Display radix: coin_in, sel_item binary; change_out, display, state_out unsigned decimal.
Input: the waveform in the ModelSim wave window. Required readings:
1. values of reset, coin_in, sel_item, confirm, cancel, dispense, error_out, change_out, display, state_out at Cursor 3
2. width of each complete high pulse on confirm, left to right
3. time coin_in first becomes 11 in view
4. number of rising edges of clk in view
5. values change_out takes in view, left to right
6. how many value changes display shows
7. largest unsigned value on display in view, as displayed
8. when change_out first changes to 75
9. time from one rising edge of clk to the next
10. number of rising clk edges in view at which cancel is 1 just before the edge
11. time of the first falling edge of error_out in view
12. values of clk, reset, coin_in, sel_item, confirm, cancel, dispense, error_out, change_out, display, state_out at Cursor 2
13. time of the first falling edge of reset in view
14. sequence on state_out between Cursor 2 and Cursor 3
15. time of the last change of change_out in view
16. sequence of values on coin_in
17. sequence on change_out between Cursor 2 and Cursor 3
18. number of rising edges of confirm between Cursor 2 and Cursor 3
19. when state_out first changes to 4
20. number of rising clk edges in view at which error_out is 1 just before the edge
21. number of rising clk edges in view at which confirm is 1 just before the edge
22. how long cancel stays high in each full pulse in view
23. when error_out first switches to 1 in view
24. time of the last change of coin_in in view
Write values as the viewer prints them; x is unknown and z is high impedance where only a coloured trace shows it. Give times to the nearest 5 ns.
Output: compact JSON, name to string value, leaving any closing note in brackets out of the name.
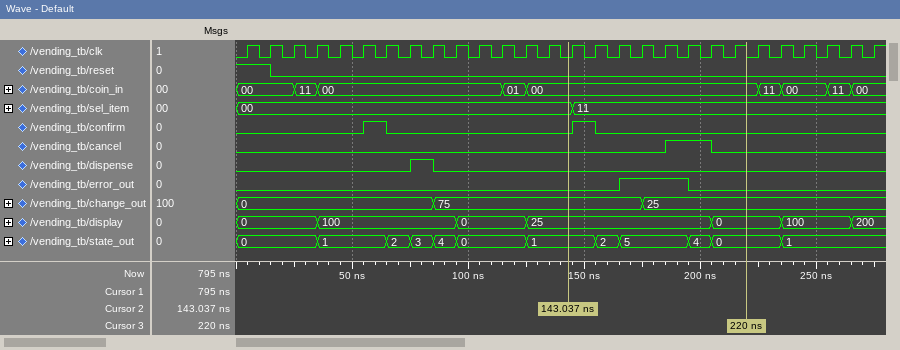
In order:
{"values of reset, coin_in, sel_item, confirm, cancel, dispense, error_out, change_out, display, state_out at Cursor 3": "reset=0, coin_in=00, sel_item=11, confirm=0, cancel=0, dispense=0, error_out=0, change_out=25, display=0, state_out=0", "width of each complete high pulse on confirm, left to right": "10 ns, 10 ns", "time coin_in first becomes 11 in view": "25 ns", "number of rising edges of clk in view": "28", "values change_out takes in view, left to right": "0, 75, 25", "how many value changes display shows": "6", "largest unsigned value on display in view, as displayed": "200", "when change_out first changes to 75": "85 ns", "time from one rising edge of clk to the next": "10 ns", "number of rising clk edges in view at which cancel is 1 just before the edge": "2", "time of the first falling edge of error_out in view": "195 ns", "values of clk, reset, coin_in, sel_item, confirm, cancel, dispense, error_out, change_out, display, state_out at Cursor 2": "clk=0, reset=0, coin_in=00, sel_item=00, confirm=0, cancel=0, dispense=0, error_out=0, change_out=75, display=25, state_out=1", "time of the first falling edge of reset in view": "15 ns", "sequence on state_out between Cursor 2 and Cursor 3": "1, 2, 5, 4, 0", "time of the last change of change_out in view": "175 ns", "sequence of values on coin_in": "00, 11, 00, 01, 00, 11, 00, 11, 00", "sequence on change_out between Cursor 2 and Cursor 3": "75, 25", "number of rising edges of confirm between Cursor 2 and Cursor 3": "1", "when state_out first changes to 4": "85 ns", "number of rising clk edges in view at which error_out is 1 just before the edge": "3", "number of rising clk edges in view at which confirm is 1 just before the edge": "2", "how long cancel stays high in each full pulse in view": "20 ns", "when error_out first switches to 1 in view": "165 ns", "time of the last change of coin_in in view": "265 ns"}
